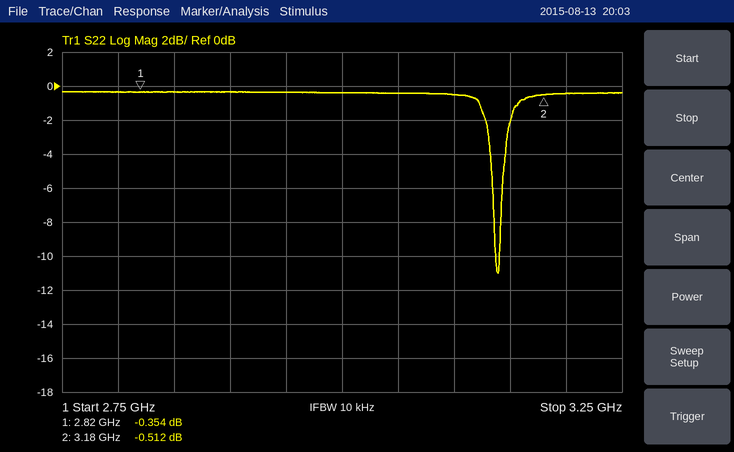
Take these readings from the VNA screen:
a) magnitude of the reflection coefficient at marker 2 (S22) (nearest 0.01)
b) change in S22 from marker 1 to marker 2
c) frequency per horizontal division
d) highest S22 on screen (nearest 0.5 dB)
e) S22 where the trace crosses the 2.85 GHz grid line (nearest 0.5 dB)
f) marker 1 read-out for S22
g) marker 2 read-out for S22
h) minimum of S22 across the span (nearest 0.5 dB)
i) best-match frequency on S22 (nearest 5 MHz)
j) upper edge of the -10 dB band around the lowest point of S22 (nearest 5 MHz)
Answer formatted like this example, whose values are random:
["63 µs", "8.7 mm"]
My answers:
["0.94", "-0.158 dB", "50 MHz", "-0.5 dB", "-0.5 dB", "-0.354 dB", "-0.512 dB", "-11.0 dB", "3.140 GHz", "3.140 GHz"]
